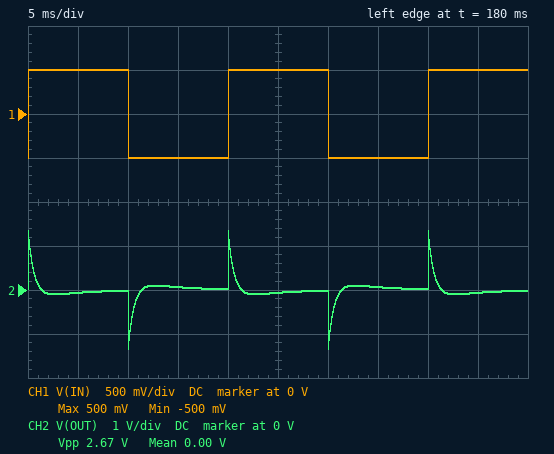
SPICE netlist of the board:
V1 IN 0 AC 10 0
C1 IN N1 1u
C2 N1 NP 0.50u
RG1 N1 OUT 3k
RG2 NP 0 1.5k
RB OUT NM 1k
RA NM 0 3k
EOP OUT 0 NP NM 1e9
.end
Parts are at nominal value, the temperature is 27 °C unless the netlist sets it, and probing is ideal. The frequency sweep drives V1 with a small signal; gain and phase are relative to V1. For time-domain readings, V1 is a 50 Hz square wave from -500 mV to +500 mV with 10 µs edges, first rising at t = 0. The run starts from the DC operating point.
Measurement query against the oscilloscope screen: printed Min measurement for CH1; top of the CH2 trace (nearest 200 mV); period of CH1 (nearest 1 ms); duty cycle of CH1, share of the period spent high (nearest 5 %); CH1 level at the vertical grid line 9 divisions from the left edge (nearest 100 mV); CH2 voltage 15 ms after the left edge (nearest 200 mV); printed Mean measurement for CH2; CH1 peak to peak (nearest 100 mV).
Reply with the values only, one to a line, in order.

-500 mV
1.4 V
20 ms
50 %
500 mV
0 V
0.00 V
1.0 V
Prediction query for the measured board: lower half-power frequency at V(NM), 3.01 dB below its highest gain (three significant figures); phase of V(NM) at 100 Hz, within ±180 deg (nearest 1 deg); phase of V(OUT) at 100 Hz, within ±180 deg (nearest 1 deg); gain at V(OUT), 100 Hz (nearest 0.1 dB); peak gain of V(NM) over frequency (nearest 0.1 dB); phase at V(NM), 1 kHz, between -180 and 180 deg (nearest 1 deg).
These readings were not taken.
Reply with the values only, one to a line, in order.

264 Hz
92 deg
92 deg
-7.1 dB
0 dB
17 deg
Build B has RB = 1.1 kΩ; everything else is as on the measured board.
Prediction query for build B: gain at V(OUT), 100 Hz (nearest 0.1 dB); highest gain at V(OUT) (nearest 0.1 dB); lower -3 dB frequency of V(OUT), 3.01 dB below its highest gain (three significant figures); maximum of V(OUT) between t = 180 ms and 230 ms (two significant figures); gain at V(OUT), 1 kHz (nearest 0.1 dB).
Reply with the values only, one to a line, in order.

-6.8 dB
2.7 dB
262 Hz
1.4 V
2.4 dB
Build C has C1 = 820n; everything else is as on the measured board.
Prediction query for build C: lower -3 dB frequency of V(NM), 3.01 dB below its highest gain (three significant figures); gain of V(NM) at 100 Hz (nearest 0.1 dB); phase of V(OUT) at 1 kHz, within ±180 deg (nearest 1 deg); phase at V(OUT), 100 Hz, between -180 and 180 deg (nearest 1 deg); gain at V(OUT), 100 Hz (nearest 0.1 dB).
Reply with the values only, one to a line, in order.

278 Hz
-10.2 dB
18 deg
97 deg
-7.7 dB
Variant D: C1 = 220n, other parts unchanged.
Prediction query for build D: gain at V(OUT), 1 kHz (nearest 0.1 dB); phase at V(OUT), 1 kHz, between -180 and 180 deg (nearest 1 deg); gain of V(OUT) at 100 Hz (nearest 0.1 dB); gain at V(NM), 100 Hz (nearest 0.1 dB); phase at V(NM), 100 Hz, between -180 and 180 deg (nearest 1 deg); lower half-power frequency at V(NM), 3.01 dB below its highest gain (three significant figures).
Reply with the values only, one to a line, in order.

1.4 dB
33 deg
-14.9 dB
-17.4 dB
124 deg
533 Hz
